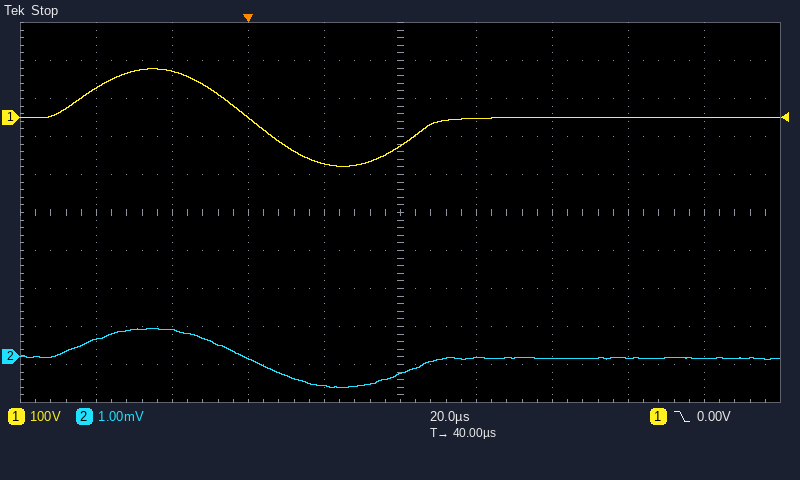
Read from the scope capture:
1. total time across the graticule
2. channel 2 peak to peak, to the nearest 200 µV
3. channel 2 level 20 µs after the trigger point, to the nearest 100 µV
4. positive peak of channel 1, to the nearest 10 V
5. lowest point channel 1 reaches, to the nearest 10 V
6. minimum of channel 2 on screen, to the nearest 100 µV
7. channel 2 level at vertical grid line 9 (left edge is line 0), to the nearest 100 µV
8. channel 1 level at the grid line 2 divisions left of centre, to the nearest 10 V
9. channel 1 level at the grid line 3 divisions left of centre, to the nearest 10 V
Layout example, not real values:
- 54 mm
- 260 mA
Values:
- 200 µs
- 1.6 mV
- -800 µV
- 130 V
- -130 V
- -800 µV
- 0.0 mV
- 0 V
- 120 V
